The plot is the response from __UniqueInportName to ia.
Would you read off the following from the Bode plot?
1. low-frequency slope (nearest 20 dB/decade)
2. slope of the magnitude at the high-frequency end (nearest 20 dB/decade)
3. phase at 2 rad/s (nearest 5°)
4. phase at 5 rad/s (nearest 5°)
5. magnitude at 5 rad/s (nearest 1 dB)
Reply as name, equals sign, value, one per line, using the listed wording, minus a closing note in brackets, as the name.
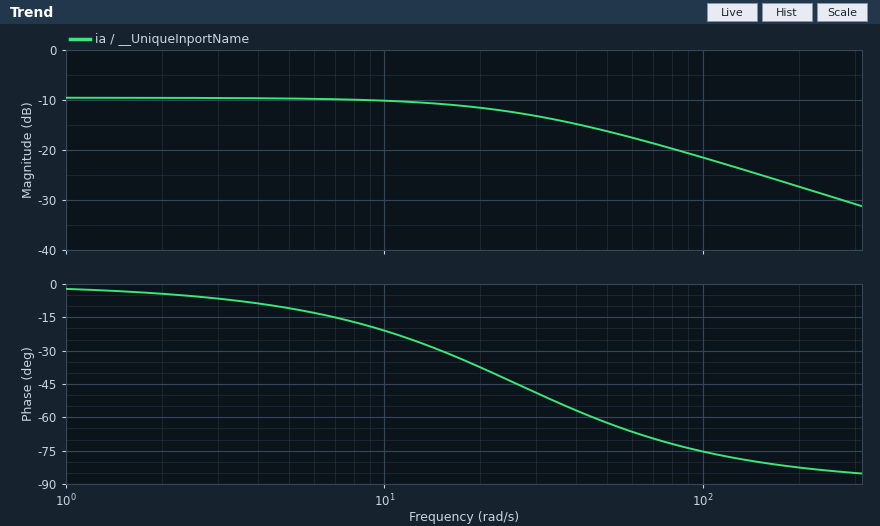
low-frequency slope = 0 dB/decade
slope of the magnitude at the high-frequency end = -20 dB/decade
phase at 2 rad/s = -5°
phase at 5 rad/s = -10°
magnitude at 5 rad/s = -10 dB
